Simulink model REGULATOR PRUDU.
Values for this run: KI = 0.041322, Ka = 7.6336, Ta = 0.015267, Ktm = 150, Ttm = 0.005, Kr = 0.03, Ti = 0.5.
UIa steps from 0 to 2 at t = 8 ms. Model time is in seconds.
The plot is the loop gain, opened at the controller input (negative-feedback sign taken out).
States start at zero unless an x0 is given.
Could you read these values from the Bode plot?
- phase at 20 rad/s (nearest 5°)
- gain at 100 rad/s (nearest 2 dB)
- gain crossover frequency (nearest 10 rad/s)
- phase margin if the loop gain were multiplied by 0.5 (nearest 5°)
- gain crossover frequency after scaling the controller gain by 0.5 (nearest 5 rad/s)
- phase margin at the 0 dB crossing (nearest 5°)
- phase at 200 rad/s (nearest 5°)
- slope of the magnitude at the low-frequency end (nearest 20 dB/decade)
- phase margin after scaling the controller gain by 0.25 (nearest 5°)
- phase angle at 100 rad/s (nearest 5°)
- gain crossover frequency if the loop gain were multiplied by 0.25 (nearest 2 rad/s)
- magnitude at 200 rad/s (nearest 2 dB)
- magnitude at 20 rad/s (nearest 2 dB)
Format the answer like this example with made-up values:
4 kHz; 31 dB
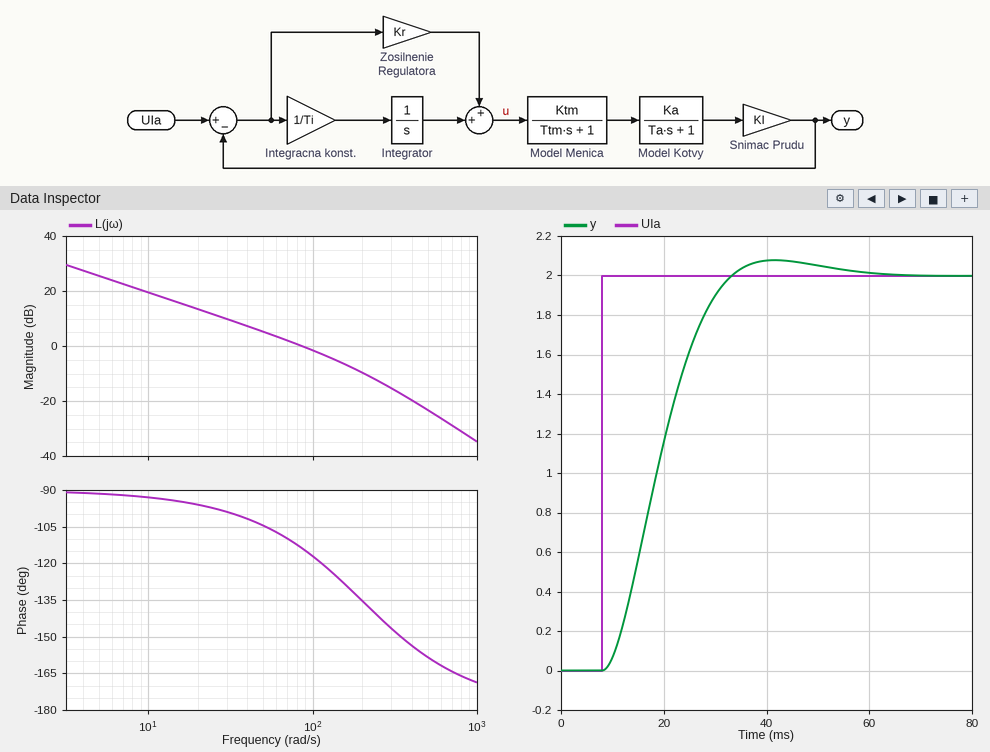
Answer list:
-95°; -2 dB; 90 rad/s; 75°; 45 rad/s; 65°; -135°; -20 dB/decade; 85°; -115°; 24 rad/s; -10 dB; 14 dB
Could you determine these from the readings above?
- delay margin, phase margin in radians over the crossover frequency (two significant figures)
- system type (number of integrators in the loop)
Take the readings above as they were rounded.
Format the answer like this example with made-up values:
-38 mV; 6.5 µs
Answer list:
0.013 s; 1
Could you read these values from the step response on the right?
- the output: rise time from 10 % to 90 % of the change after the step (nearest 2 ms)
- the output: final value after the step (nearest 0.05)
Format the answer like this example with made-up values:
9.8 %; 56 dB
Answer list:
16 ms; 2.00
